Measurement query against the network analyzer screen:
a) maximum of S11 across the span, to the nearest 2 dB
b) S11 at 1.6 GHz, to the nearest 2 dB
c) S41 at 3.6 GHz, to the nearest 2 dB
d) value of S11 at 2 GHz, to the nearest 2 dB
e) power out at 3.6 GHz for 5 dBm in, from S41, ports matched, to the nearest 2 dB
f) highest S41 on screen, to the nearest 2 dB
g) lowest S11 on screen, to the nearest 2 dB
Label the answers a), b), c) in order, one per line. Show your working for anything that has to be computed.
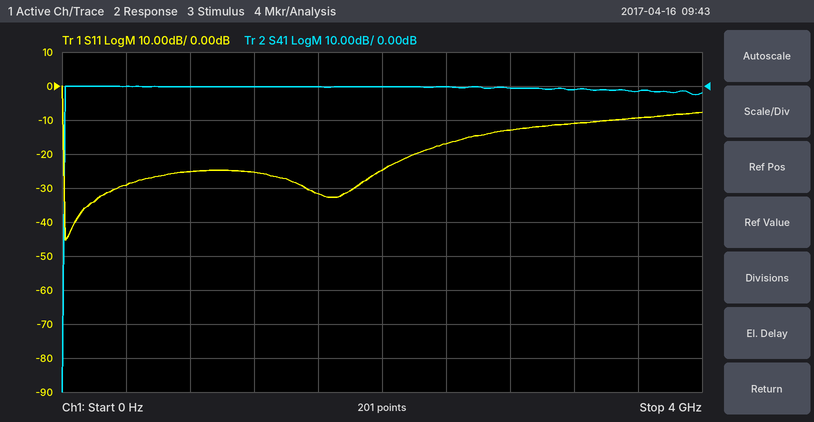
a) 0 dB
b) -32 dB
c) -2 dB
d) -24 dB
e) 5 dBm + (-2 dB) = 4 dBm
f) 0 dB
g) -46 dB
